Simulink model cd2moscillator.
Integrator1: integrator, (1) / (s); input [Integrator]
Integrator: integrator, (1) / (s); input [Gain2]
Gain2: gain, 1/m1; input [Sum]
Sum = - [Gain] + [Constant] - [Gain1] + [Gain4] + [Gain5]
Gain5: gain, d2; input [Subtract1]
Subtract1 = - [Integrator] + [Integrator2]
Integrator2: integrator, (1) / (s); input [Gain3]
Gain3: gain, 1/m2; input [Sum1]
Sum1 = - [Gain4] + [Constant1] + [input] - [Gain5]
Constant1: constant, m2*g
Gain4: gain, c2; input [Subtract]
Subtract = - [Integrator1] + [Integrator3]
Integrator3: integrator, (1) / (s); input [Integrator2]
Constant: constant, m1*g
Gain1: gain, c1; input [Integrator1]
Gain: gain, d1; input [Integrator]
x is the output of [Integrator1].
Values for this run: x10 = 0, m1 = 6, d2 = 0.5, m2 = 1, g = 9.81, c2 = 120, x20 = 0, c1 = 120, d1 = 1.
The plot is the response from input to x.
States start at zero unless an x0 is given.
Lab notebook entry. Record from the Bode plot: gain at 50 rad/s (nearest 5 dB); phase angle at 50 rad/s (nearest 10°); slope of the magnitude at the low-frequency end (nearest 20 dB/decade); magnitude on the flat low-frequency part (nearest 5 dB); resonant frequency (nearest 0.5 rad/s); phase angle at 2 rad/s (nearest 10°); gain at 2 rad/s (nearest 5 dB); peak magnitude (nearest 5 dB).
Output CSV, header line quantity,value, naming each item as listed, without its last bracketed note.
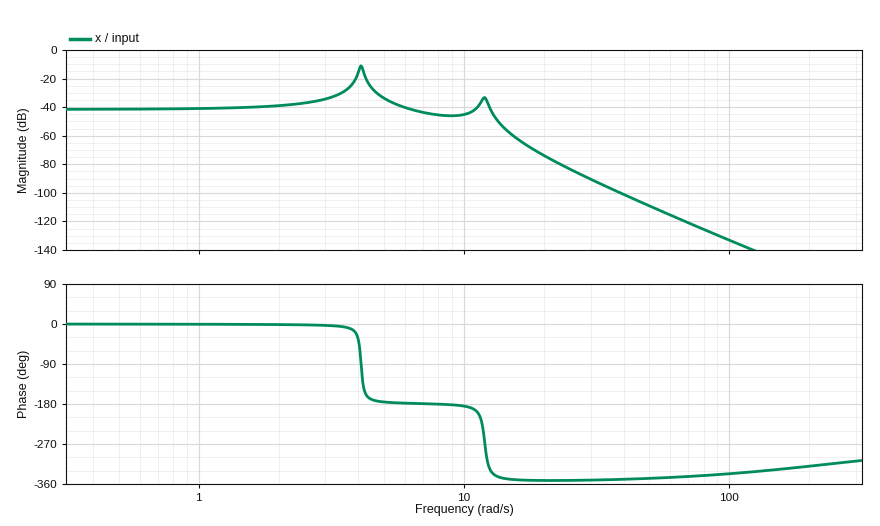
quantity,value
gain at 50 rad/s,-110 dB
phase angle at 50 rad/s,-350°
slope of the magnitude at the low-frequency end,0 dB/decade
magnitude on the flat low-frequency part,-40 dB
resonant frequency,4.0 rad/s
phase angle at 2 rad/s,0°
gain at 2 rad/s,-40 dB
peak magnitude,-10 dB
